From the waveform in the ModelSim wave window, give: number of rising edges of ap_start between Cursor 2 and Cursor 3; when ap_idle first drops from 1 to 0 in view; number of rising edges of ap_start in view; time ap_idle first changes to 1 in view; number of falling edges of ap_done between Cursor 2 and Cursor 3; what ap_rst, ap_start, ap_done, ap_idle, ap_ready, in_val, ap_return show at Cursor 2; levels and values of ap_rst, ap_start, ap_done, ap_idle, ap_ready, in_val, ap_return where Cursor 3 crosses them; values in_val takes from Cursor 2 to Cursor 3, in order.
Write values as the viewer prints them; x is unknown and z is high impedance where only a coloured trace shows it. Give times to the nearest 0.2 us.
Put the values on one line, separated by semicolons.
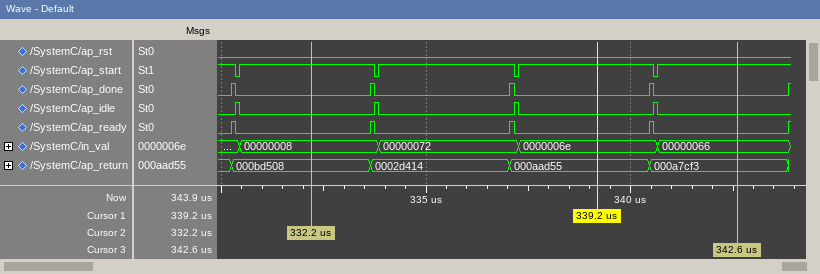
3; 330.4 us; 4; 330.4 us; 3; ap_rst=0, ap_start=1, ap_done=0, ap_idle=0, ap_ready=0, in_val=00000008, ap_return=000bd508; ap_rst=0, ap_start=1, ap_done=0, ap_idle=0, ap_ready=0, in_val=00000066, ap_return=000a7cf3; 00000008, 00000072, 0000006e, 00000066
